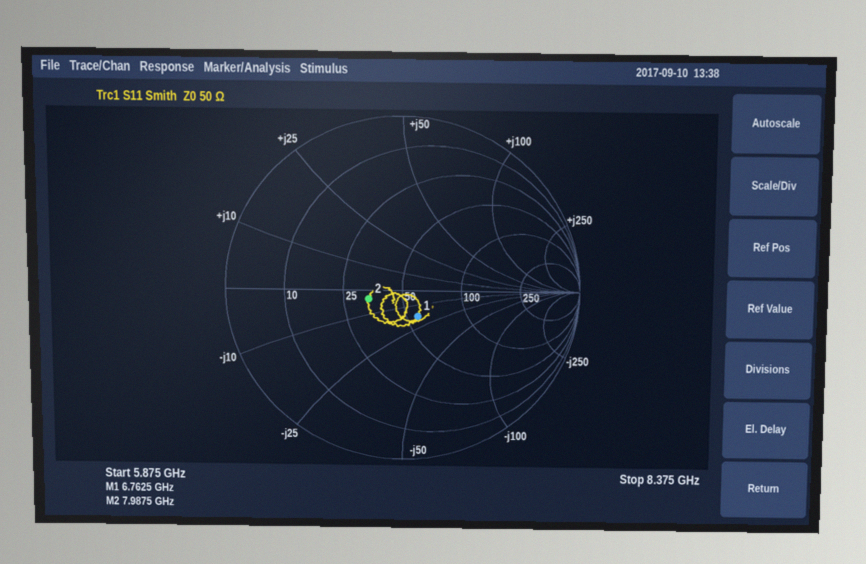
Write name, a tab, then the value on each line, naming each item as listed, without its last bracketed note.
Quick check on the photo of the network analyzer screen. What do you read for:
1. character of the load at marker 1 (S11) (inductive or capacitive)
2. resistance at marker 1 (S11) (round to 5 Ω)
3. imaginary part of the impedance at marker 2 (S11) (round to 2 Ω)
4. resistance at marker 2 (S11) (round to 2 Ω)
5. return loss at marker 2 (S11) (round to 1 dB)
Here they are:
character of the load at marker 1 (S11)	capacitive
resistance at marker 1 (S11)	55 Ω
imaginary part of the impedance at marker 2 (S11)	-4 Ω
resistance at marker 2 (S11)	34 Ω
return loss at marker 2 (S11)	14 dB
